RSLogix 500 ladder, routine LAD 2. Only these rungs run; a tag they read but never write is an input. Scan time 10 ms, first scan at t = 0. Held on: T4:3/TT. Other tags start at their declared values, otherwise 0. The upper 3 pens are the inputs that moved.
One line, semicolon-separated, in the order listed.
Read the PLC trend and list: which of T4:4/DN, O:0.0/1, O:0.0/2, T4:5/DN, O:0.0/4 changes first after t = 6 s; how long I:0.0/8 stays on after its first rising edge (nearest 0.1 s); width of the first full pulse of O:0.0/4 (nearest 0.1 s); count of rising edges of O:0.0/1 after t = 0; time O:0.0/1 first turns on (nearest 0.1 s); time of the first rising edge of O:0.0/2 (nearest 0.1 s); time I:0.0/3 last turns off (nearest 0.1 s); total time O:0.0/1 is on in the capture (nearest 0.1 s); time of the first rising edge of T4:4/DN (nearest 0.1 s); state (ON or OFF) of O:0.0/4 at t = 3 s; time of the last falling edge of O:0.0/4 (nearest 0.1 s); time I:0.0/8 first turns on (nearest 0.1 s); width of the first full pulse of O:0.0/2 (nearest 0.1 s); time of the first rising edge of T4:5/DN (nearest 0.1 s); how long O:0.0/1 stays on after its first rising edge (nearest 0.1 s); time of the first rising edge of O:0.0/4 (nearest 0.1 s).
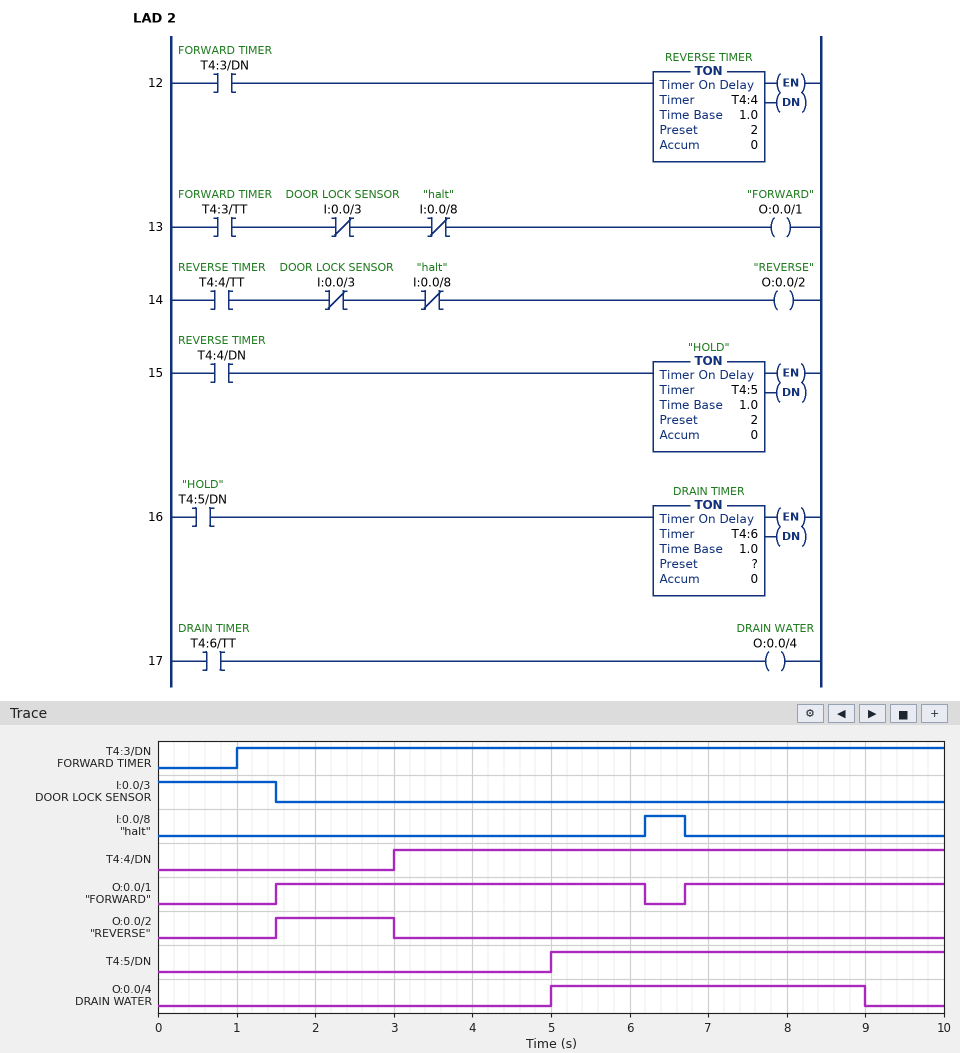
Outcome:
O:0.0/1; 0.5 s; 4.0 s; 2; 1.5 s; 1.5 s; 1.5 s; 8.0 s; 3.0 s; OFF; 9.0 s; 6.2 s; 1.5 s; 5.0 s; 4.7 s; 5.0 s
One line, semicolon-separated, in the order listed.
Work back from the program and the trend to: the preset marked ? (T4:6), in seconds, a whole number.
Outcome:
4 s
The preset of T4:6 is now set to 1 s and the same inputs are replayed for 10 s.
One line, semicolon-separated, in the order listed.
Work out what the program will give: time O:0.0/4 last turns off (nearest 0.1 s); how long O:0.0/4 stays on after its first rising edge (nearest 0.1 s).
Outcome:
6.0 s; 1.0 s
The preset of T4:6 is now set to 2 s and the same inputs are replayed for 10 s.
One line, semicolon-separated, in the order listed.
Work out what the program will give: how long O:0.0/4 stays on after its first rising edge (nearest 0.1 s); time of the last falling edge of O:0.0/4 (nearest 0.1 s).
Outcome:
2.0 s; 7.0 s
